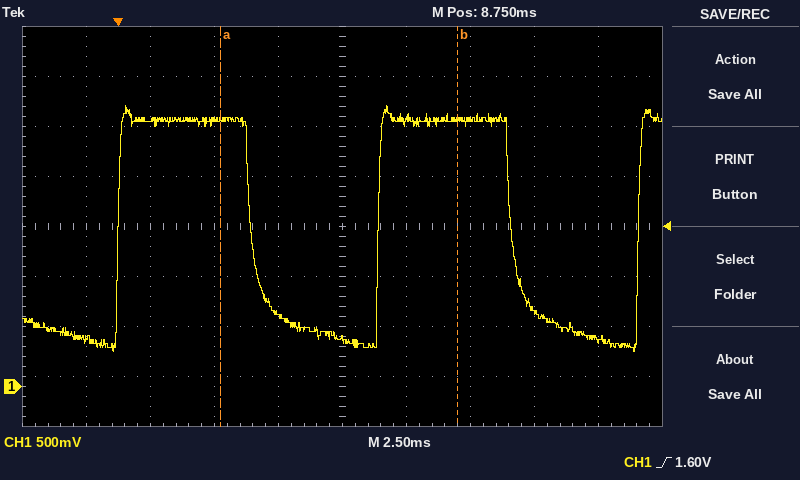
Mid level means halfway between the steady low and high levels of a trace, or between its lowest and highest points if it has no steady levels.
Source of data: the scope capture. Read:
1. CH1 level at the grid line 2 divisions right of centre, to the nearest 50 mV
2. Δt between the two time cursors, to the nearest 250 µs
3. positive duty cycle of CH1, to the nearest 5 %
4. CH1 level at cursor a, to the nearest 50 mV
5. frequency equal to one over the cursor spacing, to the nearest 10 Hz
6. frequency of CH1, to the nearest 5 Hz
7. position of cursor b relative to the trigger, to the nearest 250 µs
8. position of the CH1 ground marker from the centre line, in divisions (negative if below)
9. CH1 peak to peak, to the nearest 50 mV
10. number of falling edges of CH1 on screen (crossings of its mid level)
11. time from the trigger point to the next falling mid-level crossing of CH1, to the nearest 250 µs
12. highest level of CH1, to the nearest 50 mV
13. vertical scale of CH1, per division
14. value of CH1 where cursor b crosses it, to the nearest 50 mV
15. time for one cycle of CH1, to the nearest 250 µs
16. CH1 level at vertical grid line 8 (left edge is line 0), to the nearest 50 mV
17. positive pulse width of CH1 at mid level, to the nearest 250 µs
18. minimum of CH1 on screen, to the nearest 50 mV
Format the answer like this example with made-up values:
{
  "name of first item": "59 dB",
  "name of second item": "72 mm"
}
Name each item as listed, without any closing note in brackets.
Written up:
{
  "CH1 level at the grid line 2 divisions right of centre, to the nearest 50 mV": "2.65 V",
  "Δt between the two time cursors, to the nearest 250 µs": "9.25 ms",
  "positive duty cycle of CH1, to the nearest 5 %": "50 %",
  "CH1 level at cursor a, to the nearest 50 mV": "2.65 V",
  "frequency equal to one over the cursor spacing, to the nearest 10 Hz": "110 Hz",
  "frequency of CH1, to the nearest 5 Hz": "100 Hz",
  "position of cursor b relative to the trigger, to the nearest 250 µs": "+13.25 ms",
  "position of the CH1 ground marker from the centre line, in divisions": "-3.2 div",
  "CH1 peak to peak, to the nearest 50 mV": "2.45 V",
  "number of falling edges of CH1 on screen": "2",
  "time from the trigger point to the next falling mid-level crossing of CH1, to the nearest 250 µs": "5.25 ms",
  "highest level of CH1, to the nearest 50 mV": "2.80 V",
  "vertical scale of CH1, per division": "500 mV",
  "value of CH1 where cursor b crosses it, to the nearest 50 mV": "2.65 V",
  "time for one cycle of CH1, to the nearest 250 µs": "10.25 ms",
  "CH1 level at vertical grid line 8 (left edge is line 0), to the nearest 50 mV": "750 mV",
  "positive pulse width of CH1 at mid level, to the nearest 250 µs": "5.25 ms",
  "minimum of CH1 on screen, to the nearest 50 mV": "350 mV"
}
